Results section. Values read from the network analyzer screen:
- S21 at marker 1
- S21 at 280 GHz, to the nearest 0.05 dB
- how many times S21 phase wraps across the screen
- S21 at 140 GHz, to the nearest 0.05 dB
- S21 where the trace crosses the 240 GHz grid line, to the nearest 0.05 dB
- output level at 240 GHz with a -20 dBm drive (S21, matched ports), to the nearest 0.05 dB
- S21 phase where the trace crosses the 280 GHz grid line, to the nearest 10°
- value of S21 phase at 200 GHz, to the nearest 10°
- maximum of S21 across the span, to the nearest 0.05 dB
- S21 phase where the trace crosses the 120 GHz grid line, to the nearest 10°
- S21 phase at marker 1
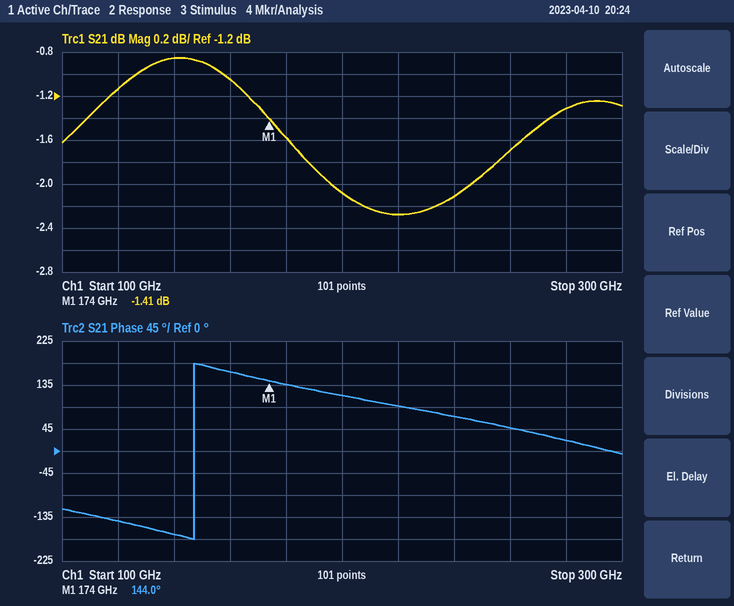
-1.41 dB
-1.30 dB
1
-0.85 dB
-2.10 dB
-22.10 dBm
20°
110°
-0.85 dB
-140°
144.0°
